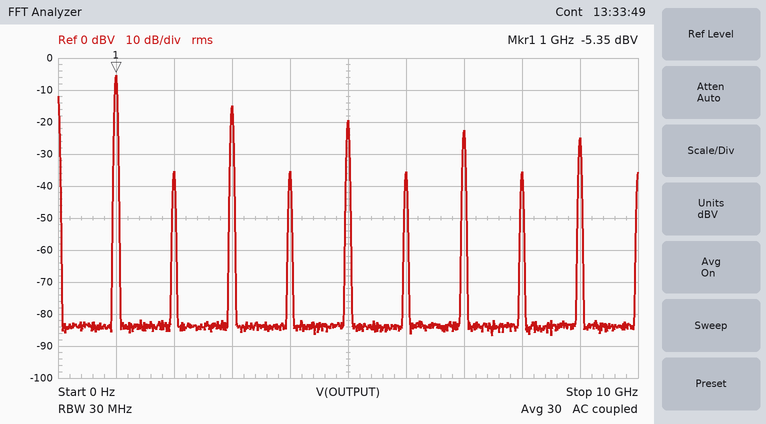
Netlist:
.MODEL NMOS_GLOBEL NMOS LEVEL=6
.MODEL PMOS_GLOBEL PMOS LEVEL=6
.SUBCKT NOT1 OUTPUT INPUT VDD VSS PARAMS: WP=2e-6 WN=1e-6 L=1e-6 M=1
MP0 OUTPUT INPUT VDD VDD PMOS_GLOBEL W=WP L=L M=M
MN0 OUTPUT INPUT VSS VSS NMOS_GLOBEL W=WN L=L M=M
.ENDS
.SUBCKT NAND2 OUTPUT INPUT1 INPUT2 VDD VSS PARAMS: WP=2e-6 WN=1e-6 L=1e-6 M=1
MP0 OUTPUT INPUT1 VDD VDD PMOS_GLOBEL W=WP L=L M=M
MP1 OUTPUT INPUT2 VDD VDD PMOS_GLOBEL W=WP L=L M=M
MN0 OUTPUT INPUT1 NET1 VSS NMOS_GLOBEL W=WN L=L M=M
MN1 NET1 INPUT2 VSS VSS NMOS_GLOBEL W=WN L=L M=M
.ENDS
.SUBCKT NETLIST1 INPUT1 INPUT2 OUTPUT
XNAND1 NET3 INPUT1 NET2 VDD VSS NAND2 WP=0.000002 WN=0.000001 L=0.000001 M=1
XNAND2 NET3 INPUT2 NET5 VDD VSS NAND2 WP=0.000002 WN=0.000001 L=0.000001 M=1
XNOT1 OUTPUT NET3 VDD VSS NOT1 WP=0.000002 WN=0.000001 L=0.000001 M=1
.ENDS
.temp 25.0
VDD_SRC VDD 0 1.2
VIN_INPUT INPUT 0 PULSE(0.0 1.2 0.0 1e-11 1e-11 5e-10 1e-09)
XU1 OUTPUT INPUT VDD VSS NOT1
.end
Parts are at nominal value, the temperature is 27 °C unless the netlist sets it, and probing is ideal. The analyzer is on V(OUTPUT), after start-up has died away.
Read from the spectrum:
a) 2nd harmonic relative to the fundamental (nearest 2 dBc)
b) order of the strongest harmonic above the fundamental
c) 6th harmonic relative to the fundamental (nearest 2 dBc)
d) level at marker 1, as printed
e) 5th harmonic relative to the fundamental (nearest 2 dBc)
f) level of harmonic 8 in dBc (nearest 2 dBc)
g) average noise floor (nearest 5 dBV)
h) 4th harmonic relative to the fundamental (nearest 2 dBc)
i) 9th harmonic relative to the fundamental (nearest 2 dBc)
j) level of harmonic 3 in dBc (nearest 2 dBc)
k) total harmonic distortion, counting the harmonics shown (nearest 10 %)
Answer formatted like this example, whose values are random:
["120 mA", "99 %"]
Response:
["-30 dBc", "3", "-30 dBc", "-5.35 dBV", "-14 dBc", "-30 dBc", "-85 dBV", "-30 dBc", "-20 dBc", "-10 dBc", "40 %"]
